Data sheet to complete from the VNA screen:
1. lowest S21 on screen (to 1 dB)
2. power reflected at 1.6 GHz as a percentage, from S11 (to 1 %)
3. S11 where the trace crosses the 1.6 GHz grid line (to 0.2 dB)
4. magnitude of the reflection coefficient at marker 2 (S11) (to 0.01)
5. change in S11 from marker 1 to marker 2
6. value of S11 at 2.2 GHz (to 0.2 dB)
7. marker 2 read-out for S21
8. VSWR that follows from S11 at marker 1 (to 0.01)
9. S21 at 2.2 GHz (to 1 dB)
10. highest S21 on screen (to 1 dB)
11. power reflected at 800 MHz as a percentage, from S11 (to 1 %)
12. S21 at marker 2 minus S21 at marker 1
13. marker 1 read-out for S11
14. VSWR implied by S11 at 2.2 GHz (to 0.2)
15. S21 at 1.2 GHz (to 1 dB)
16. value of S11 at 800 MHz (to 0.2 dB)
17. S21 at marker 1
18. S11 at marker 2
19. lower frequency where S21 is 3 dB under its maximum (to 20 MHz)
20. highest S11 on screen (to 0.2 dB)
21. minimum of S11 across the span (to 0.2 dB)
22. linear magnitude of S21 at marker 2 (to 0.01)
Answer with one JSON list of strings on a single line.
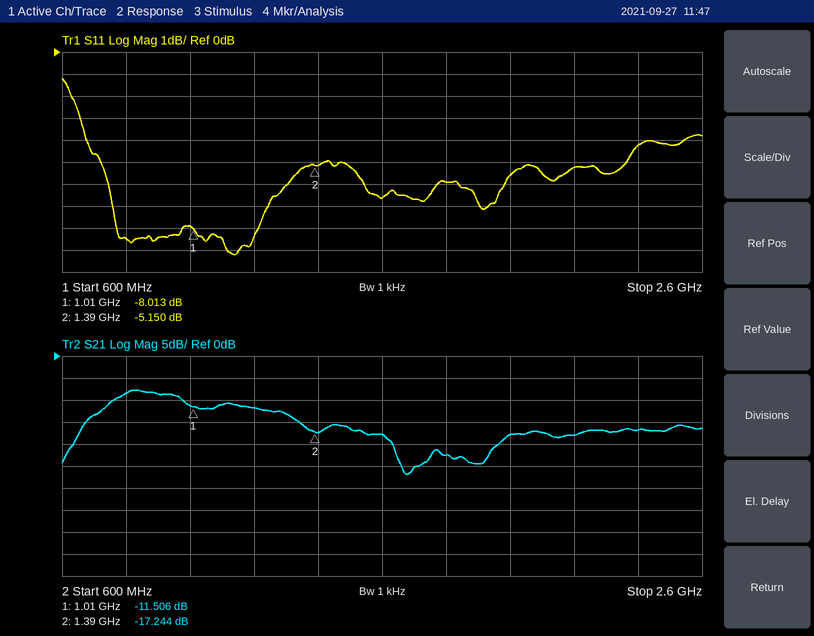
["-27 dB", "22 %", "-6.6 dB", "0.55", "2.863 dB", "-5.2 dB", "-17.244 dB", "2.32", "-18 dB", "-8 dB", "14 %", "-5.738 dB", "-8.013 dB", "3.4", "-12 dB", "-8.4 dB", "-11.506 dB", "-5.150 dB", "740 MHz", "-1.2 dB", "-9.2 dB", "0.14"]
